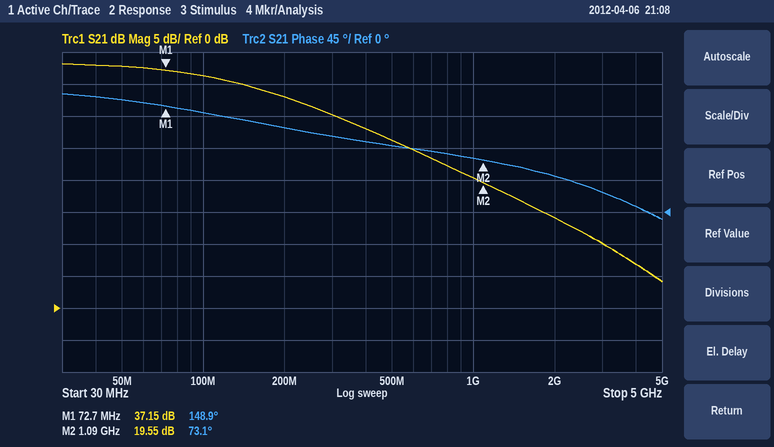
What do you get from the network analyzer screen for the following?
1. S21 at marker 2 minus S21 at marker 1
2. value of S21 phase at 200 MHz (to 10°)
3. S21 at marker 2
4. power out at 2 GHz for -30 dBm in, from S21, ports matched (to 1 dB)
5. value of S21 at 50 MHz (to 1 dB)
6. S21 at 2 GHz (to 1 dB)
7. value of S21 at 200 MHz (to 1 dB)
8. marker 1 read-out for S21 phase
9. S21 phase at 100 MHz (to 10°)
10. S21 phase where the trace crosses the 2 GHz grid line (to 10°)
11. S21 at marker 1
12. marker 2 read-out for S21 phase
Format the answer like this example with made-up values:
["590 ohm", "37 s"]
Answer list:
["-17.60 dB", "120°", "19.55 dB", "-16 dBm", "38 dB", "14 dB", "33 dB", "148.9°", "140°", "50°", "37.15 dB", "73.1°"]
